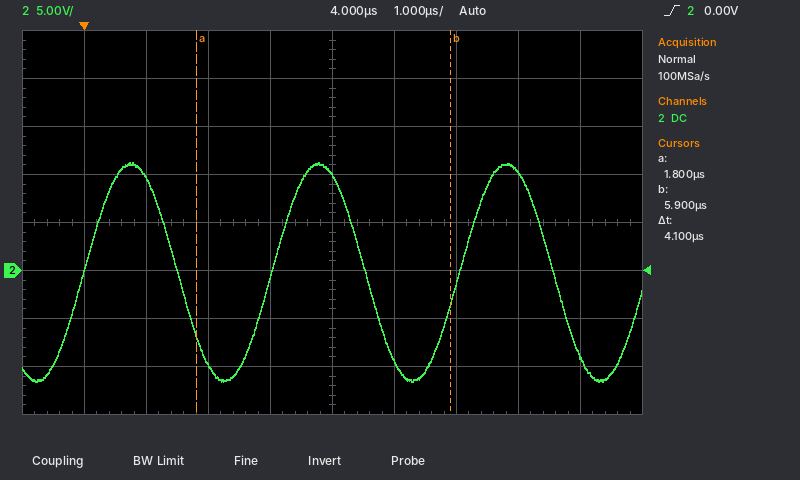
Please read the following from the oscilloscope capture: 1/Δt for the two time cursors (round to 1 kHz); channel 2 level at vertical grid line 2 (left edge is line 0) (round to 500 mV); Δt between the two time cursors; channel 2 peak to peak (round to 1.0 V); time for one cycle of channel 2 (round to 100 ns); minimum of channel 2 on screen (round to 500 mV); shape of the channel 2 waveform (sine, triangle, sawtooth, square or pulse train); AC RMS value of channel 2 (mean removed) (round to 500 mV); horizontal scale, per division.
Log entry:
244 kHz
9.5 V
4.1 µs
23.0 V
3.0 µs
-11.5 V
sine
8.0 V
1 µs
